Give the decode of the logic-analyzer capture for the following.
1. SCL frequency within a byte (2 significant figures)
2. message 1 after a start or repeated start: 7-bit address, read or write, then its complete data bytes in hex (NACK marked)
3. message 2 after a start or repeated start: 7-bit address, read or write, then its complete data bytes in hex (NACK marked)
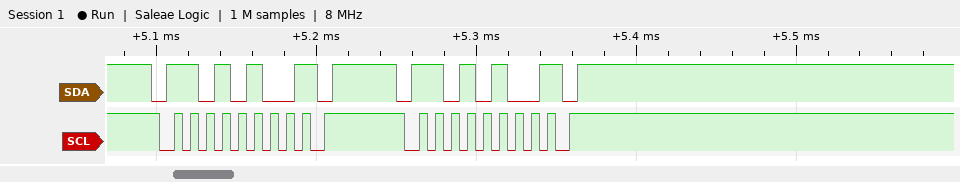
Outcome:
100 kHz
0x6A write NACK
0x6A write NACK
